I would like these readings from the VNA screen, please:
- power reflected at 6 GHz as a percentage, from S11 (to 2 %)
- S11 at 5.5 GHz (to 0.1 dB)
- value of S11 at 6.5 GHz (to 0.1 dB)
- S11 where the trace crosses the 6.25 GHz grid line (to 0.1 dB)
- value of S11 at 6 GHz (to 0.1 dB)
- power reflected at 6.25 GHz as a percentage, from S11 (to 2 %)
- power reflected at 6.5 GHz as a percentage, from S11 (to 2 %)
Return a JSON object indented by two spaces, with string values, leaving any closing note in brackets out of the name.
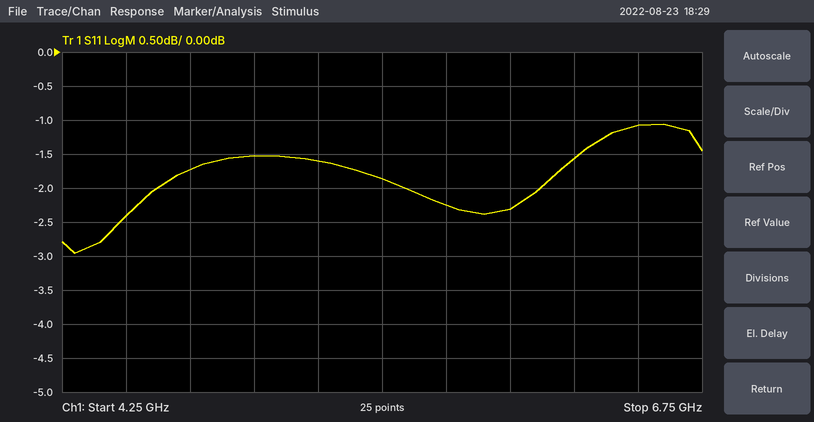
{
  "power reflected at 6 GHz as a percentage, from S11": "58 %",
  "S11 at 5.5 GHz": "-1.9 dB",
  "value of S11 at 6.5 GHz": "-1.1 dB",
  "S11 where the trace crosses the 6.25 GHz grid line": "-1.6 dB",
  "value of S11 at 6 GHz": "-2.3 dB",
  "power reflected at 6.25 GHz as a percentage, from S11": "70 %",
  "power reflected at 6.5 GHz as a percentage, from S11": "78 %"
}
